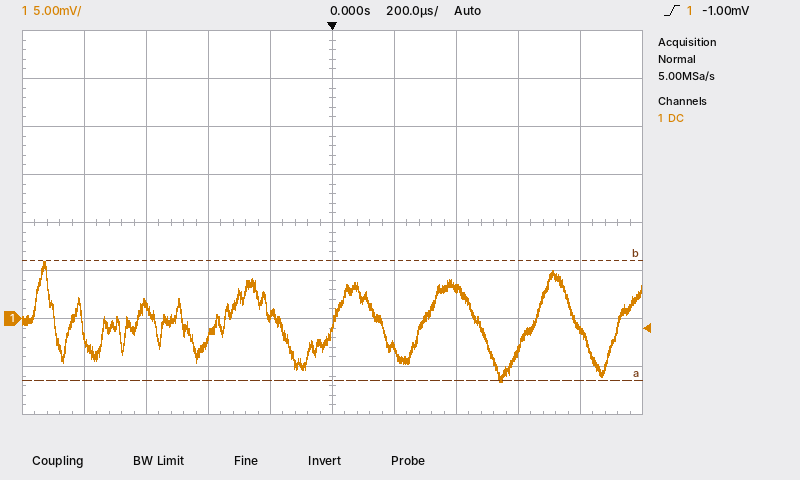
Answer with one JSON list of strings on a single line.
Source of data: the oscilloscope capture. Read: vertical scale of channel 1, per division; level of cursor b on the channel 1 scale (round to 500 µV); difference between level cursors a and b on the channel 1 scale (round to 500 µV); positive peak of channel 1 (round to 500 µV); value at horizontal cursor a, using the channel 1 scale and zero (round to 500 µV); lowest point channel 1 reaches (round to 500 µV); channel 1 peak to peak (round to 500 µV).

["5 mV", "6.0 mV", "12.5 mV", "6.0 mV", "-6.5 mV", "-6.5 mV", "12.5 mV"]
